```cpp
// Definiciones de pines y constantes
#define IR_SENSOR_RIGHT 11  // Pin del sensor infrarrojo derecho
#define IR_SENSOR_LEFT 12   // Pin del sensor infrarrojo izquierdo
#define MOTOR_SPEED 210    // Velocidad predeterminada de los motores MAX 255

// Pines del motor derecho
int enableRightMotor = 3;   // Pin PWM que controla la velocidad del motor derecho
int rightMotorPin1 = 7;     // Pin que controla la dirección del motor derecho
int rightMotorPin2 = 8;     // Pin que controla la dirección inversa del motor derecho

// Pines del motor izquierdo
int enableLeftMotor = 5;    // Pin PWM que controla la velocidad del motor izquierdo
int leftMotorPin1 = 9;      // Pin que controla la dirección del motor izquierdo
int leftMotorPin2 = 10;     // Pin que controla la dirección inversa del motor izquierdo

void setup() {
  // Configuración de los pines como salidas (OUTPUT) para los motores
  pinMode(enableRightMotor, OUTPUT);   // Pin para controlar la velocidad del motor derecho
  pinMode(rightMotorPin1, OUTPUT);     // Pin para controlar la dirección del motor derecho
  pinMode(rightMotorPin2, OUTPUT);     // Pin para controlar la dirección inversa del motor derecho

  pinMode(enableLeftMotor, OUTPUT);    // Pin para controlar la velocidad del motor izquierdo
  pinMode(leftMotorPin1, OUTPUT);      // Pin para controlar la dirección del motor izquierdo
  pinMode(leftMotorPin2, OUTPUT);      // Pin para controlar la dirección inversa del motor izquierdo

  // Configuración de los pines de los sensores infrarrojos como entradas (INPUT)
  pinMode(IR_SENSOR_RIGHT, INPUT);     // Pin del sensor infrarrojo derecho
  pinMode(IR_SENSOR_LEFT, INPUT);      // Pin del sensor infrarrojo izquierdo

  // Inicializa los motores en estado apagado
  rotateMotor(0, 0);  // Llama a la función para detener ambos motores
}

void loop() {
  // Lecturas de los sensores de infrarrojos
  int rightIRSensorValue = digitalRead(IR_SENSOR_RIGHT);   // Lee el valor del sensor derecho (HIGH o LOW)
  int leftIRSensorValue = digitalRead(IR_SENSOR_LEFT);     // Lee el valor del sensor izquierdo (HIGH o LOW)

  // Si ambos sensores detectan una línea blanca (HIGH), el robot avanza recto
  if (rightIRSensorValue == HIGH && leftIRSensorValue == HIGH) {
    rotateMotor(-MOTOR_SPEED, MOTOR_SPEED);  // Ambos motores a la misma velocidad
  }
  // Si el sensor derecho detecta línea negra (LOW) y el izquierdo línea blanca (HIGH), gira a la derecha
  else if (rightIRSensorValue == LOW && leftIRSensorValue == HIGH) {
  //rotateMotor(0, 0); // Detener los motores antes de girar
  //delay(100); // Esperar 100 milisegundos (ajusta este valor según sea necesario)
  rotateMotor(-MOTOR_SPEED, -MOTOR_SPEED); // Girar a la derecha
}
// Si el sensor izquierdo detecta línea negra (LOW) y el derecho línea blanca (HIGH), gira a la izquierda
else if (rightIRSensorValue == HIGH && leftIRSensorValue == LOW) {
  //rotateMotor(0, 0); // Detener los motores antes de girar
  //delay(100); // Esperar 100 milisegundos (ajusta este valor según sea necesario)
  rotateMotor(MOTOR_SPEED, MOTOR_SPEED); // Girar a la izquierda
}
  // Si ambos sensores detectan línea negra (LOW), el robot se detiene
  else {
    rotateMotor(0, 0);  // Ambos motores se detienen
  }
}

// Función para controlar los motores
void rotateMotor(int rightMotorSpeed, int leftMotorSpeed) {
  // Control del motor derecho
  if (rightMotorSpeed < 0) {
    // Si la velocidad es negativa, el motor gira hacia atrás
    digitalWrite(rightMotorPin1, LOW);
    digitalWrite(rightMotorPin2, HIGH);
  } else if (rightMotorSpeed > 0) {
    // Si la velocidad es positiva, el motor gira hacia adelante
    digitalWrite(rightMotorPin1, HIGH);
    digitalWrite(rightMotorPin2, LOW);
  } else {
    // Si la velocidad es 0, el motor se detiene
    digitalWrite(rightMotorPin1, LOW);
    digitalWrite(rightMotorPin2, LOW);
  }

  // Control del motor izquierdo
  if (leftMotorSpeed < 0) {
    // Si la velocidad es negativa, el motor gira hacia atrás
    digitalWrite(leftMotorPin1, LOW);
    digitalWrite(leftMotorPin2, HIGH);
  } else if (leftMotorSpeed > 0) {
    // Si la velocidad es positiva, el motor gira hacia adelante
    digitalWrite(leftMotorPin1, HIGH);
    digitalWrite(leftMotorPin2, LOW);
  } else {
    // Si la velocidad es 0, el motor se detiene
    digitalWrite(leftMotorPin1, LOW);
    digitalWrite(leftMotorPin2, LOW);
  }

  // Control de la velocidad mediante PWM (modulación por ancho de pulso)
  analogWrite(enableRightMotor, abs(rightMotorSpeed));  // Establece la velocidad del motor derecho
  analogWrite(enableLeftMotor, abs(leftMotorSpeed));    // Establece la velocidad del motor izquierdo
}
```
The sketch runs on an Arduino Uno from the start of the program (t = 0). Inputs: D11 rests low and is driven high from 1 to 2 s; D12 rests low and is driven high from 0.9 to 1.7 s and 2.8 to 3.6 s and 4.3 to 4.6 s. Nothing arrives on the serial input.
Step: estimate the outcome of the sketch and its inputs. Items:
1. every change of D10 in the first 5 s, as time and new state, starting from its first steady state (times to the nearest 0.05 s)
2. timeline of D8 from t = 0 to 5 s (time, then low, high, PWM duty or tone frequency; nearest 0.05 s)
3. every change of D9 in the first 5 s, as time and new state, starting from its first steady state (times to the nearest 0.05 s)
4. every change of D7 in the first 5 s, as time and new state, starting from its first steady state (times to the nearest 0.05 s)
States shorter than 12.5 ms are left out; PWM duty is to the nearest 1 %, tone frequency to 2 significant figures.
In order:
0 s low; 0.9 s high; 1 s low; 2.8 s high; 3.6 s low; 4.3 s high; 4.6 s low
0 s low; 0.9 s high; 1.7 s low; 2.8 s high; 3.6 s low; 4.3 s high; 4.6 s low
0 s low; 1 s high; 2 s low
0 s low; 1.7 s high; 2 s low
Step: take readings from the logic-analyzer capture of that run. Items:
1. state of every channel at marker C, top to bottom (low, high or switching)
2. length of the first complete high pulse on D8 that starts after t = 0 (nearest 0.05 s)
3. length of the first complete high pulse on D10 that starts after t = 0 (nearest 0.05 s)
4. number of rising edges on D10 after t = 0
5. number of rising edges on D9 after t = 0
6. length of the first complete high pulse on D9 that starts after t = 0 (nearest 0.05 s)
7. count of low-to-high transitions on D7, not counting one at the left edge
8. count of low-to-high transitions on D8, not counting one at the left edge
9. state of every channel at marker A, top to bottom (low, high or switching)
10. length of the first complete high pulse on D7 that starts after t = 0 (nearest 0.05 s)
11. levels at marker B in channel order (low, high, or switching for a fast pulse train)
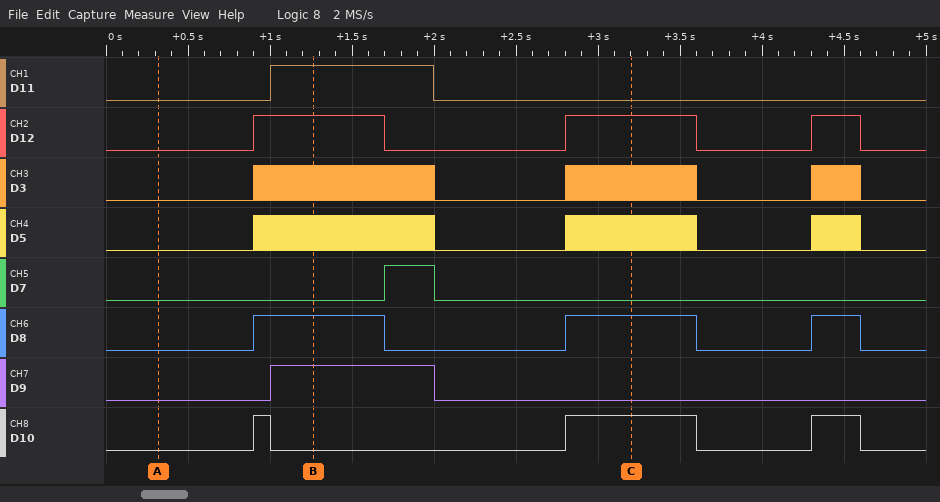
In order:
D11 low, D12 high, D3 switching, D5 switching, D7 low, D8 high, D9 low, D10 high
0.80 s
0.10 s
3
1
1.00 s
1
3
D11 low, D12 low, D3 low, D5 low, D7 low, D8 low, D9 low, D10 low
0.30 s
D11 high, D12 high, D3 switching, D5 switching, D7 low, D8 high, D9 high, D10 low
